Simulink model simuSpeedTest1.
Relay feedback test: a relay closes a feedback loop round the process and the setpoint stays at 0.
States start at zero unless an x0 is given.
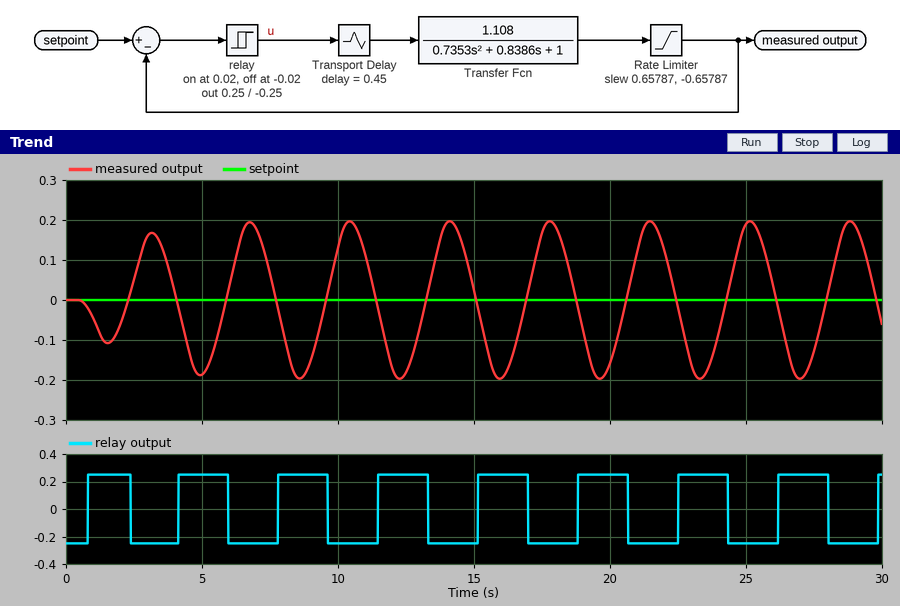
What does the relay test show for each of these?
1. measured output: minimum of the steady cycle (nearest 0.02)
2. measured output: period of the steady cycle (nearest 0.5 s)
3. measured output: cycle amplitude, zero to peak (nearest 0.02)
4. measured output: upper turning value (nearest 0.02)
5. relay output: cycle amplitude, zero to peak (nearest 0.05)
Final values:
-0.20
3.5 s
0.20
0.20
0.25
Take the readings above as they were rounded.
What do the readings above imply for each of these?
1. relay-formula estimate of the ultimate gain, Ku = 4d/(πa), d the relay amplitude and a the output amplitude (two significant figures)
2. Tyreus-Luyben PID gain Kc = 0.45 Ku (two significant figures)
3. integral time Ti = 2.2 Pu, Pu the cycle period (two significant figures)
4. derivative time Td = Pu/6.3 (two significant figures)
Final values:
1.6
0.72
7.7 s
0.56 s
